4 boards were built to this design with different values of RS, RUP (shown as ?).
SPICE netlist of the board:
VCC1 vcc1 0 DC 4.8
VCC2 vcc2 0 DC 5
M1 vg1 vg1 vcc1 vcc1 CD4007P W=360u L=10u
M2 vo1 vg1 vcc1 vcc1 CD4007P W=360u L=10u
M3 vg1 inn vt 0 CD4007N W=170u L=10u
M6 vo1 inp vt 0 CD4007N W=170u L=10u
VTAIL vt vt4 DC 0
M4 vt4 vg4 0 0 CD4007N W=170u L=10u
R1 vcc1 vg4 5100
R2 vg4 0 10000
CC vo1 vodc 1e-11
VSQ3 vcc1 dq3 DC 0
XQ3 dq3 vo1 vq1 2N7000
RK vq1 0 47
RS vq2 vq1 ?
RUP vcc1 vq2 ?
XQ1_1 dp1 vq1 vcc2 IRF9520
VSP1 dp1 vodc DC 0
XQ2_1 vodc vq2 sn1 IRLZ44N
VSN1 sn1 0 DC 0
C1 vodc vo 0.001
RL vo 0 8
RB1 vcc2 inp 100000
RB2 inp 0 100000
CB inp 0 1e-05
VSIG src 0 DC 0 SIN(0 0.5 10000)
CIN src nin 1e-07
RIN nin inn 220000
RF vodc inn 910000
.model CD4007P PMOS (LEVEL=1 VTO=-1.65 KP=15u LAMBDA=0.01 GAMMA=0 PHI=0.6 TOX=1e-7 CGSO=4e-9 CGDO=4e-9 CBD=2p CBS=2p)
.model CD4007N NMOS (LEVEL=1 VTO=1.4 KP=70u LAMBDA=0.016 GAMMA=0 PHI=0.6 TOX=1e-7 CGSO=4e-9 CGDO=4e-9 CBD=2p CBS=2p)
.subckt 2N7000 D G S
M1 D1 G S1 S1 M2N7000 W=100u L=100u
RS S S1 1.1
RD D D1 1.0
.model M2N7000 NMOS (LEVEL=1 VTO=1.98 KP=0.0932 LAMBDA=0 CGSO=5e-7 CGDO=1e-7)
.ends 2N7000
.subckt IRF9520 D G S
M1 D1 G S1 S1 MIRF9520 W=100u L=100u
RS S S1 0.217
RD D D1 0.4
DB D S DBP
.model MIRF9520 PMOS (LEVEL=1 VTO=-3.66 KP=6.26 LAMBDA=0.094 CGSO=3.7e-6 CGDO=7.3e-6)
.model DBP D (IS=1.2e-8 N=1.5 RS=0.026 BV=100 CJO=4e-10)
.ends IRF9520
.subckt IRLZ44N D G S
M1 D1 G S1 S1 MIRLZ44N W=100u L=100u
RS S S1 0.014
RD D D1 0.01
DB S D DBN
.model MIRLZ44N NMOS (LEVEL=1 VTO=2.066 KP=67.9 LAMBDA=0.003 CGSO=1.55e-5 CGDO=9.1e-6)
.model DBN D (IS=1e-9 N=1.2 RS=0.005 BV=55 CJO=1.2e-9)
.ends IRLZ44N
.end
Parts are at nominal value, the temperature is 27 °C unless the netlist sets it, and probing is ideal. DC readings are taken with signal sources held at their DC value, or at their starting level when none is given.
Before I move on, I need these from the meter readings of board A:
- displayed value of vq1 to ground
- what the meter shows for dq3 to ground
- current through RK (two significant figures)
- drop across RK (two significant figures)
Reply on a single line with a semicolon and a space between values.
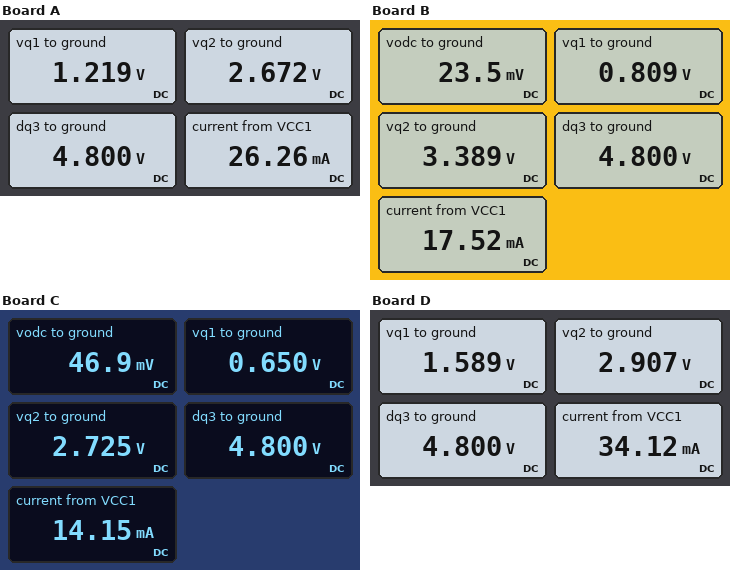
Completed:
1.219 V; 4.800 V; 26 mA; 1.2 V
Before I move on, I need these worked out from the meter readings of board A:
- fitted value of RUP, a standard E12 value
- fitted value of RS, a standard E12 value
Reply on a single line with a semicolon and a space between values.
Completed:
82 Ω; 56 Ω
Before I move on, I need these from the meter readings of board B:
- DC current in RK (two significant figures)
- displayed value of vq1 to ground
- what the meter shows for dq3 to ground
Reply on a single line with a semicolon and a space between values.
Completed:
17 mA; 0.809 V; 4.800 V
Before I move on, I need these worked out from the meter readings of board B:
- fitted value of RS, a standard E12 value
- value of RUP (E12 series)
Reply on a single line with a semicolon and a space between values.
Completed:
150 Ω; 82 Ω
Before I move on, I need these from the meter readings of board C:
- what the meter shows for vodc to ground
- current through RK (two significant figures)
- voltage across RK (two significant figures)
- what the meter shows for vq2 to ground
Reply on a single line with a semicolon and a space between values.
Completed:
46.9 mV; 14 mA; 650 mV; 2.725 V
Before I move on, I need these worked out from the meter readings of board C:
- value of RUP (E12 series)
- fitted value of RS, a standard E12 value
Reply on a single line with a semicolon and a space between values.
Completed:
150 Ω; 150 Ω
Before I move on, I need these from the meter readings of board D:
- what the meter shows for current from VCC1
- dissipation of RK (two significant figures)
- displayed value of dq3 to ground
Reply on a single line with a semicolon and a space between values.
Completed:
34.12 mA; 54 mW; 4.800 V
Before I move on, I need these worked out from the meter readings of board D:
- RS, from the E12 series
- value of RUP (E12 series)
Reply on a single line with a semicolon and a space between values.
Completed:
39 Ω; 56 Ω
